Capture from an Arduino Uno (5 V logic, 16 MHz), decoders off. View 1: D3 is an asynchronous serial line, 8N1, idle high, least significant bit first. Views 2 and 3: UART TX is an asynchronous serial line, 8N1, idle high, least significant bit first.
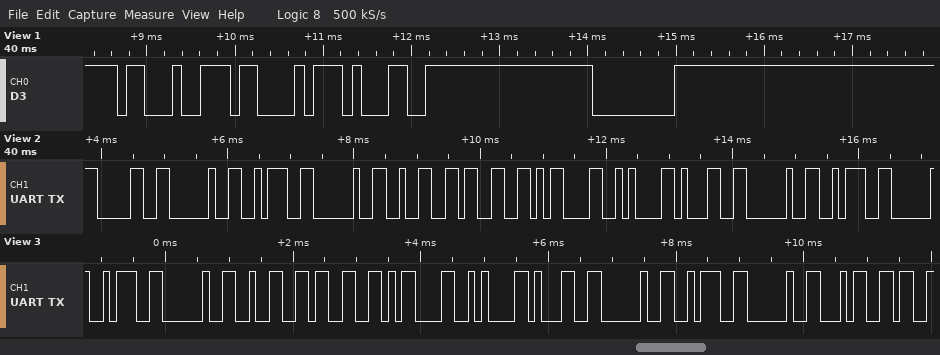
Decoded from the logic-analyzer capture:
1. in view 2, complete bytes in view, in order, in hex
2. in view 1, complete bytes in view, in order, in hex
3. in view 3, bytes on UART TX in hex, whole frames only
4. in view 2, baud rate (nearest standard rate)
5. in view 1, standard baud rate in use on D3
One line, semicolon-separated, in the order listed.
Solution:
30 20 3A 20 32 33 0D 0A 31 20 3A; 23 43 31 00; 3A 20 32 33 0D 0A 31 20 3A 20 34; 9600 baud; 9600 baud
